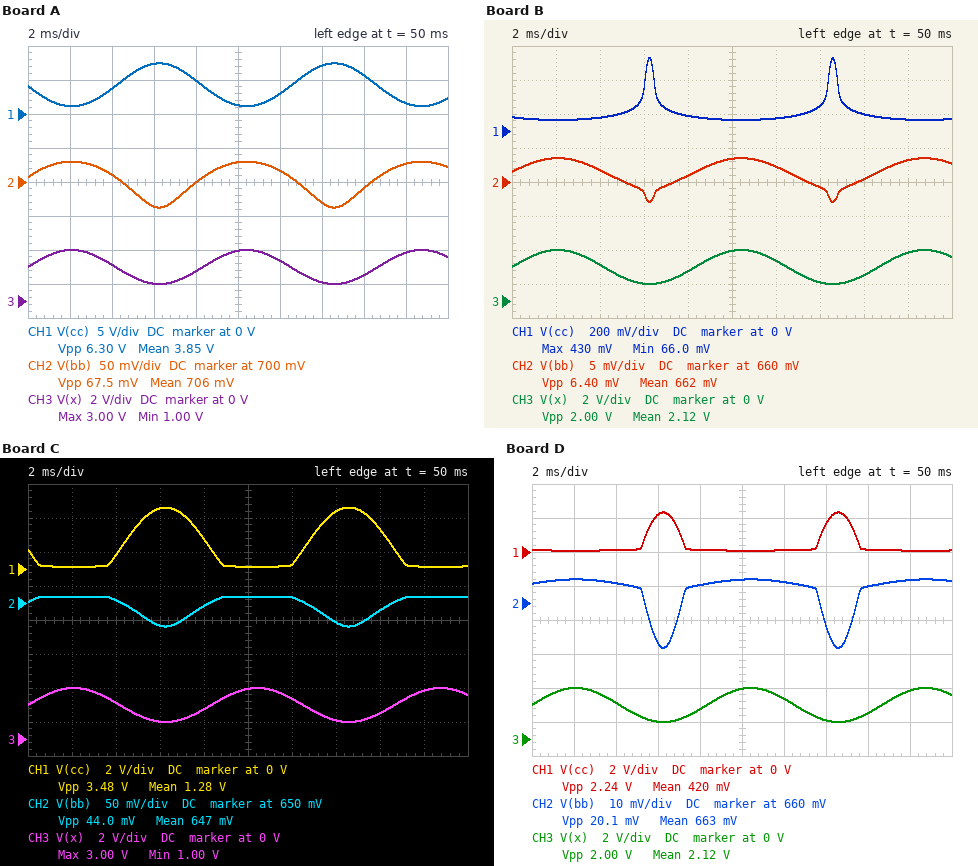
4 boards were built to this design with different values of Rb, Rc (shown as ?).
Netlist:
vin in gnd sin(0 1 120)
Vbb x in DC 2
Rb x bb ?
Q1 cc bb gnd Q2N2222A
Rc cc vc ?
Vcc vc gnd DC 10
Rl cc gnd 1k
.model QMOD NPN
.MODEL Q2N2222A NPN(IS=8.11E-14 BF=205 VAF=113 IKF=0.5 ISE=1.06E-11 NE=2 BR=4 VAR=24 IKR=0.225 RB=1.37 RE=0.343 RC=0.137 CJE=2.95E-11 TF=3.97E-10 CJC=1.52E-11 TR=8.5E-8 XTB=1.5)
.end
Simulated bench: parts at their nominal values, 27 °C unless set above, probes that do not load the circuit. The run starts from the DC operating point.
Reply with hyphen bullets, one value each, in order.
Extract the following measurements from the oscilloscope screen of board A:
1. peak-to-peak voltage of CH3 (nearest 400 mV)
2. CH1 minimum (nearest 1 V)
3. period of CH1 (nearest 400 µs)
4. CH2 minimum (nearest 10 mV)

- 2.0 V
- 1 V
- 8.4 ms
- 660 mV
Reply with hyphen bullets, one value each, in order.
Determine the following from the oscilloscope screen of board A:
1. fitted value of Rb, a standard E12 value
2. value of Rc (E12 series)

- 6.8 kΩ
- 150 Ω
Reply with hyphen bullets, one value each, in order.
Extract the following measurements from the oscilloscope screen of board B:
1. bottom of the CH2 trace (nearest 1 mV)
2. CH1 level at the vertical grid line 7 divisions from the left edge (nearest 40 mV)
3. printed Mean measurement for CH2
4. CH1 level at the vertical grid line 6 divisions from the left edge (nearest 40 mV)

- 657 mV
- 160 mV
- 662 mV
- 80 mV
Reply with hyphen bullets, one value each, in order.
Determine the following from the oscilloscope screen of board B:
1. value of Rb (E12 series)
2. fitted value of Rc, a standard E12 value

- 8.2 kΩ
- 1.2 kΩ
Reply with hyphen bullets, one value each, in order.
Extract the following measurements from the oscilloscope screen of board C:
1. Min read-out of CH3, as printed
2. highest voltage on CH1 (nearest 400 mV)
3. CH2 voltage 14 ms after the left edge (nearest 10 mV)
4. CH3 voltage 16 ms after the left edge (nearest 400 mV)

- 1.00 V
- 3.6 V
- 620 mV
- 1.6 V
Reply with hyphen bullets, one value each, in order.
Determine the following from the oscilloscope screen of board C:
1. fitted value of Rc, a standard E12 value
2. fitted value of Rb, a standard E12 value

- 1.2 kΩ
- 39 kΩ
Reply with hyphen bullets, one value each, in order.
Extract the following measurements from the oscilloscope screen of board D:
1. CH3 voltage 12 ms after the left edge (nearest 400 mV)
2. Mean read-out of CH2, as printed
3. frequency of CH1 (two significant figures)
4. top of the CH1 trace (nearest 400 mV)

- 2.4 V
- 663 mV
- 120 Hz
- 2.4 V
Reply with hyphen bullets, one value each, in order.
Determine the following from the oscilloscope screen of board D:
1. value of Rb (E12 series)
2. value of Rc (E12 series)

- 12 kΩ
- 1 kΩ
